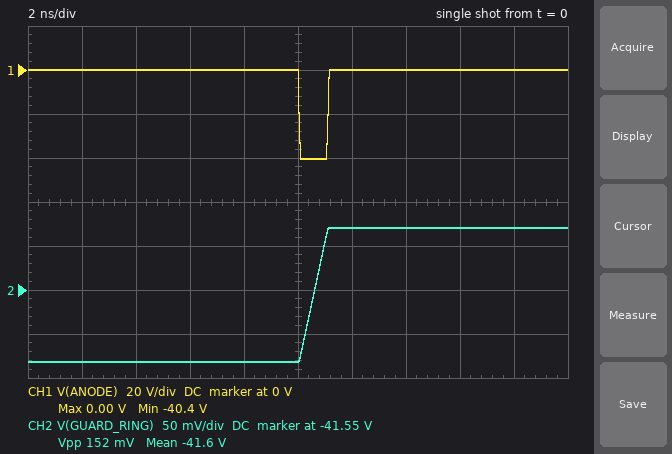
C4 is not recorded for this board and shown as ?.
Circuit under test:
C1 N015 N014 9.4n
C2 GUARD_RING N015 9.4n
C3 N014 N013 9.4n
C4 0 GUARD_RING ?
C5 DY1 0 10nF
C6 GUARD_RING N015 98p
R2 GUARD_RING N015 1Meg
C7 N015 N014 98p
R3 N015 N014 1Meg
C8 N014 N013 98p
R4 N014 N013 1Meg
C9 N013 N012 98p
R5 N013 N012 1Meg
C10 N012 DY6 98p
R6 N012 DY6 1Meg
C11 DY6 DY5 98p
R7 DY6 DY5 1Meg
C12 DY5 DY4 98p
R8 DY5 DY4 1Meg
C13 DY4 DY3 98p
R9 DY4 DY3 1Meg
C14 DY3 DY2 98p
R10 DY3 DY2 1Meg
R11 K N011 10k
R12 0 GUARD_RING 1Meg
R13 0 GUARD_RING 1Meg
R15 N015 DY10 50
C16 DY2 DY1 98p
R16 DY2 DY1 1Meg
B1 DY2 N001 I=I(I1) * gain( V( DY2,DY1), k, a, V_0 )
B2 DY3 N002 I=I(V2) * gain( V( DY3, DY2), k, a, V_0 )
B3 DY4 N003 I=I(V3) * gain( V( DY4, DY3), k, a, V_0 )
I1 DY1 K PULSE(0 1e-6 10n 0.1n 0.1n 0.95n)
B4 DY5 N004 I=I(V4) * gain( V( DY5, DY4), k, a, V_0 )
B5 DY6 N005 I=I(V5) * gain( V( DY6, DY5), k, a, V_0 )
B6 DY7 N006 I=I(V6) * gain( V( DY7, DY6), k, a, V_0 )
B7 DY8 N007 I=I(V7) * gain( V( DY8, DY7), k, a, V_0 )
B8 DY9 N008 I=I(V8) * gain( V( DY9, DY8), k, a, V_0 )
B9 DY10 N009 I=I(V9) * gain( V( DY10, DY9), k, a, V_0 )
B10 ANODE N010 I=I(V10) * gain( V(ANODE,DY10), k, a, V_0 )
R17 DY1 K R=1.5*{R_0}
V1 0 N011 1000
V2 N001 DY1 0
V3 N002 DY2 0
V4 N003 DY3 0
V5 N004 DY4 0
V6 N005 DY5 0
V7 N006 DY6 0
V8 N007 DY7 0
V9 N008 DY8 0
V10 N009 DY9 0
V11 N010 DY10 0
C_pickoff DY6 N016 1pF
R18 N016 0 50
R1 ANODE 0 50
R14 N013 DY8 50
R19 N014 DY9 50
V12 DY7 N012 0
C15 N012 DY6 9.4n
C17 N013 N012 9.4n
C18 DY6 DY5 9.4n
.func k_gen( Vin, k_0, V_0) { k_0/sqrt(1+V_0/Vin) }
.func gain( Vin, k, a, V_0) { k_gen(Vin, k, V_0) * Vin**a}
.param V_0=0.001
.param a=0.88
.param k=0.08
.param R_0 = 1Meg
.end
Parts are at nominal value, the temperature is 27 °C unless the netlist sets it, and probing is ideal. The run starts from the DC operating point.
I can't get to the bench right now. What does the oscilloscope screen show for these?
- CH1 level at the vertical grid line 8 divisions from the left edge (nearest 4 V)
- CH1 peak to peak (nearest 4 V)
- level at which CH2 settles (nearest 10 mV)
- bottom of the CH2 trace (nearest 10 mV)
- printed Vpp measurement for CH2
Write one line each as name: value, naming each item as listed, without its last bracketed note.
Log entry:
CH1 level at the vertical grid line 8 divisions from the left edge: 0 V
CH1 peak to peak: 40 V
level at which CH2 settles: -41.48 V
bottom of the CH2 trace: -41.63 V
printed Vpp measurement for CH2: 152 mV
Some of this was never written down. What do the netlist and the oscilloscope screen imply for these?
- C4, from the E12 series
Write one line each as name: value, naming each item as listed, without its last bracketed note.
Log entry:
C4, from the E12 series: 5.6 nF
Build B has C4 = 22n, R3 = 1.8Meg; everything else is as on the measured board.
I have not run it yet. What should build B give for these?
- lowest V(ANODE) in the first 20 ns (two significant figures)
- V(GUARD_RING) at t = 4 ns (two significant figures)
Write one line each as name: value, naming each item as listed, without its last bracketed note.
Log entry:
lowest V(ANODE) in the first 20 ns: -37 V
V(GUARD_RING) at t = 4 ns: -39 V
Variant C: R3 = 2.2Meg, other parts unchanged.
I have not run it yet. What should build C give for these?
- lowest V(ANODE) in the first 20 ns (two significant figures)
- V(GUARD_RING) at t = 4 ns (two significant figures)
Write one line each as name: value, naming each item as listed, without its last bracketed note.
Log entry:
lowest V(ANODE) in the first 20 ns: -34 V
V(GUARD_RING) at t = 4 ns: -38 V
